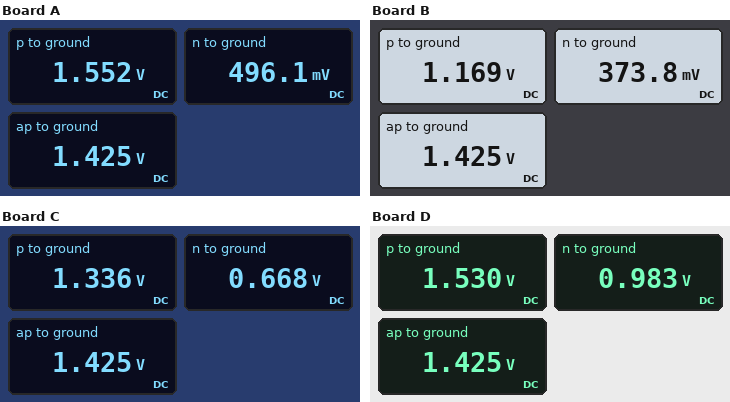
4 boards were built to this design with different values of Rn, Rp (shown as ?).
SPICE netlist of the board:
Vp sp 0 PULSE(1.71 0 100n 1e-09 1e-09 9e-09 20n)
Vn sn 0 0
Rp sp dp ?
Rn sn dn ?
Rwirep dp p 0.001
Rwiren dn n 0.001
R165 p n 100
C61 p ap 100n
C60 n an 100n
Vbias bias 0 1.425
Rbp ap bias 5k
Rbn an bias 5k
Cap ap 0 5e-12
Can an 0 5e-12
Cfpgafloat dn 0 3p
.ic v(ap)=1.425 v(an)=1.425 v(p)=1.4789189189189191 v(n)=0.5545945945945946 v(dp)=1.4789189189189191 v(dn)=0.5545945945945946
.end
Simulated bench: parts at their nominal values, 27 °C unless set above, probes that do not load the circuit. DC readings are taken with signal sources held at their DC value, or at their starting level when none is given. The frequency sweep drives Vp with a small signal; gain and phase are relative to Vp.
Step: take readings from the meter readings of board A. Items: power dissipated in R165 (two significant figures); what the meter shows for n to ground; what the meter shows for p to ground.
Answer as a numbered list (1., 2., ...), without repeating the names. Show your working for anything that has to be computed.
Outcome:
1. (1.552 V - 496.1 mV)^2 / 100 Ω = 11 mW
2. 496.1 mV
3. 1.552 V
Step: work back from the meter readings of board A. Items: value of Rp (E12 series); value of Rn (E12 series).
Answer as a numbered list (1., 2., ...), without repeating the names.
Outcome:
1. 15 Ω
2. 47 Ω
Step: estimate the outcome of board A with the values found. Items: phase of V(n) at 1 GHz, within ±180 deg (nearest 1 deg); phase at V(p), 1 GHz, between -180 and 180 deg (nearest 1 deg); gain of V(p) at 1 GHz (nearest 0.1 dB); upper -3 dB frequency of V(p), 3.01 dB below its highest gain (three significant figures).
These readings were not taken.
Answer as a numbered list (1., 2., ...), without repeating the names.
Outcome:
1. -81 deg
2. -23 deg
3. -1.9 dB
4. 2.22 GHz
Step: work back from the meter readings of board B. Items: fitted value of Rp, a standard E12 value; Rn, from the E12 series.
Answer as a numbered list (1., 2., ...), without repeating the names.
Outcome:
1. 68 Ω
2. 47 Ω
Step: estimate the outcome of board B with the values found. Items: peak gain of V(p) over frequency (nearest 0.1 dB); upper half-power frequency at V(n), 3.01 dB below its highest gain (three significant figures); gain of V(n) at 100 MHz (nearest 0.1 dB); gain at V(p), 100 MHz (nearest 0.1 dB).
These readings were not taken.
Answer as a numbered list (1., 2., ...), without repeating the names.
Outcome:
1. -3.4 dB
2. 381 MHz
3. -13.6 dB
4. -3.5 dB
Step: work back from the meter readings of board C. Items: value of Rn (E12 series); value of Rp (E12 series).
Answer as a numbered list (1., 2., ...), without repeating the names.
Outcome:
1. 100 Ω
2. 56 Ω
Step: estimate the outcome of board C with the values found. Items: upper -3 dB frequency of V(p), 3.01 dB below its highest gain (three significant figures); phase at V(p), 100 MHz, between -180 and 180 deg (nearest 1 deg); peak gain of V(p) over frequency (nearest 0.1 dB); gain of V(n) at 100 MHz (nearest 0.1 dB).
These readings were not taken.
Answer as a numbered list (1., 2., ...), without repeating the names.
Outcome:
1. 542 MHz
2. -10 deg
3. -2.2 dB
4. -8.9 dB
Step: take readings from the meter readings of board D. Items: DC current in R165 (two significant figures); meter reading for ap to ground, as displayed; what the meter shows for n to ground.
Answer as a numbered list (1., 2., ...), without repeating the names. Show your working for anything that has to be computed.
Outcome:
1. (1.53 V - 983 mV) / 100 Ω = 5.5 mA
2. 1.425 V
3. 0.983 V
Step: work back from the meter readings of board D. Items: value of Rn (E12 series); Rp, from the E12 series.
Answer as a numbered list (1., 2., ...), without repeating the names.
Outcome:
1. 180 Ω
2. 33 Ω
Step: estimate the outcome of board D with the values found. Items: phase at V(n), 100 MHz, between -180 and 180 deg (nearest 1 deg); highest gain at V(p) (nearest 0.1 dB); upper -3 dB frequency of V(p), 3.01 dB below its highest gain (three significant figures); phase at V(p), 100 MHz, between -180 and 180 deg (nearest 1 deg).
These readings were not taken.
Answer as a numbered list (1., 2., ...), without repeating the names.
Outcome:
1. -26 deg
2. -1.0 dB
3. 809 MHz
4. -8 deg
